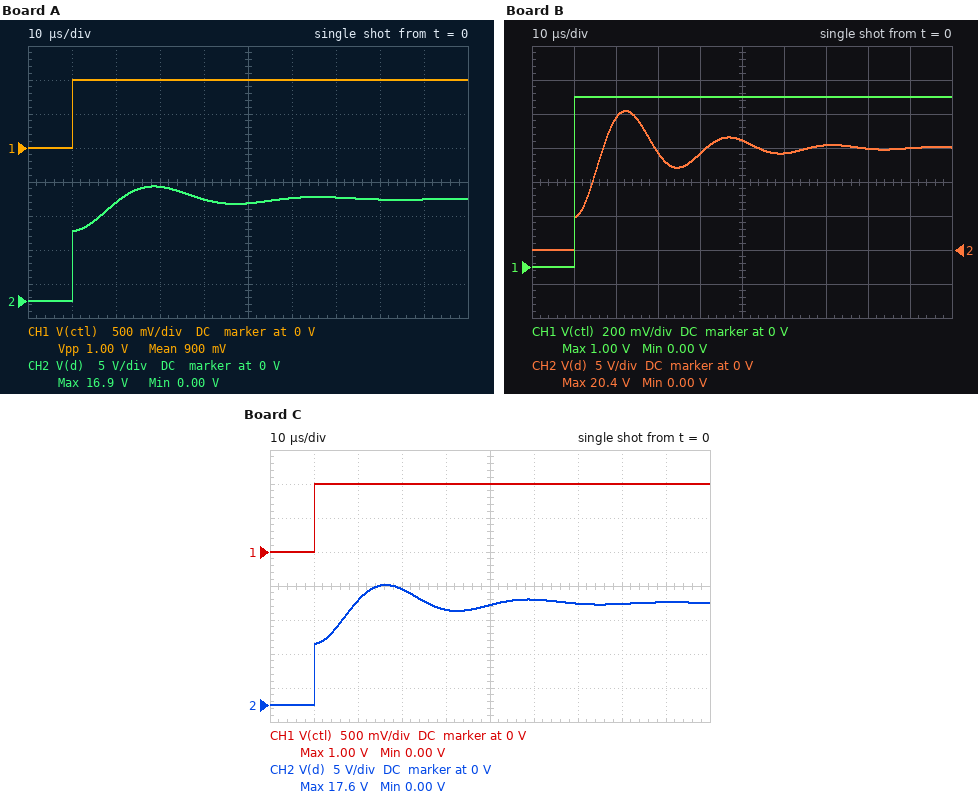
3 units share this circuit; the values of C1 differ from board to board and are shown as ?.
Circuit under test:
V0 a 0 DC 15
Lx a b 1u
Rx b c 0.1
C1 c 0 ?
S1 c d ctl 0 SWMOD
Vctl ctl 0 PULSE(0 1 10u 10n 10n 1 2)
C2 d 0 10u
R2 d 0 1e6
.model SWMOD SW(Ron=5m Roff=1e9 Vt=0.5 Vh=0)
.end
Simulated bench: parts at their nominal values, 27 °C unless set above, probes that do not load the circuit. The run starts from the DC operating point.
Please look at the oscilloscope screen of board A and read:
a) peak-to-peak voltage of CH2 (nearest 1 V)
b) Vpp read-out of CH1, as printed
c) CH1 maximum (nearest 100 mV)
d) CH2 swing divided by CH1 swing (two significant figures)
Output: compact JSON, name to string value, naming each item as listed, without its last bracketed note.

{"peak-to-peak voltage of CH2": "17 V", "Vpp read-out of CH1, as printed": "1.00 V", "CH1 maximum": "1.0 V", "CH2 swing divided by CH1 swing": "17"}
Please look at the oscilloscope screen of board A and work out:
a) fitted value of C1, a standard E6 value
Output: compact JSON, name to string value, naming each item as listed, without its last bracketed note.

{"fitted value of C1, a standard E6 value": "22 µF"}
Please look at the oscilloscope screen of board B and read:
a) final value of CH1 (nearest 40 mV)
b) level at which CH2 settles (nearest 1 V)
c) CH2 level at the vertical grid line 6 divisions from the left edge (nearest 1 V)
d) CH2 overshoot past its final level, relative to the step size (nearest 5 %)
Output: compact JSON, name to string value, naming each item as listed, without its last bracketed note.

{"final value of CH1": "1.00 V", "level at which CH2 settles": "15 V", "CH2 level at the vertical grid line 6 divisions from the left edge": "14 V", "CH2 overshoot past its final level, relative to the step size": "35 %"}
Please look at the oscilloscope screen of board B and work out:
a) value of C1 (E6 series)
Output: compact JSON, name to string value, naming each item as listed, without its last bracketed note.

{"value of C1": "4.7 µF"}
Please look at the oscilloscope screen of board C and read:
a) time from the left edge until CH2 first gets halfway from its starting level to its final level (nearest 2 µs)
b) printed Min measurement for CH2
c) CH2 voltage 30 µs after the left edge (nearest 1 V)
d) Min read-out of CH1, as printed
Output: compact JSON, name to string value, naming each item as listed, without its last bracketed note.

{"time from the left edge until CH2 first gets halfway from its starting level to its final level": "10 µs", "printed Min measurement for CH2": "0.00 V", "CH2 voltage 30 µs after the left edge": "17 V", "Min read-out of CH1, as printed": "0.00 V"}
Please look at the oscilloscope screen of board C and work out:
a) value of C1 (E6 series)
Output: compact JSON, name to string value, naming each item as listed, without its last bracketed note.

{"value of C1": "15 µF"}
